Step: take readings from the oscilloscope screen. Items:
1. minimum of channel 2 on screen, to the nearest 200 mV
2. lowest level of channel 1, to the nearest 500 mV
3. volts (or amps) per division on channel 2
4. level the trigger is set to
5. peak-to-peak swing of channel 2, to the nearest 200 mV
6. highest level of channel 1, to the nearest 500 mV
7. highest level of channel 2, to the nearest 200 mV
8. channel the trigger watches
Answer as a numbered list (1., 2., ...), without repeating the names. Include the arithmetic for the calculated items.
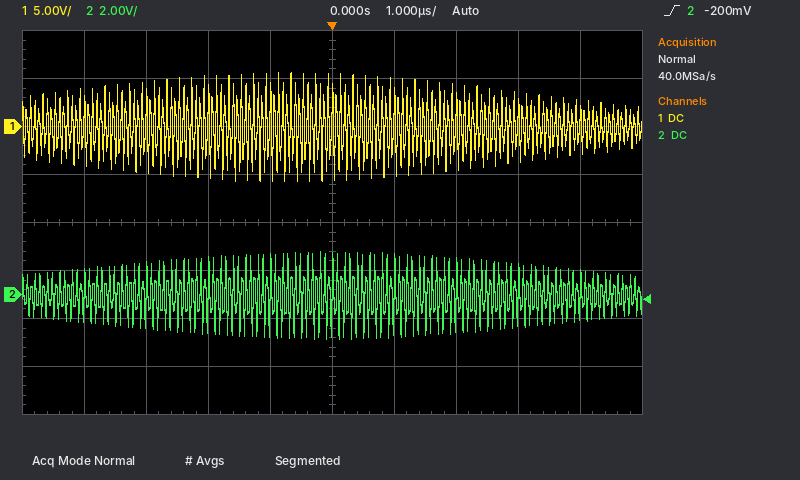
1. -1.8 V
2. -5.5 V
3. 2 V
4. -200 mV
5. 1.8 V − (-1.8 V) = 3.6 V
6. 5.5 V
7. 1.8 V
8. channel 2
